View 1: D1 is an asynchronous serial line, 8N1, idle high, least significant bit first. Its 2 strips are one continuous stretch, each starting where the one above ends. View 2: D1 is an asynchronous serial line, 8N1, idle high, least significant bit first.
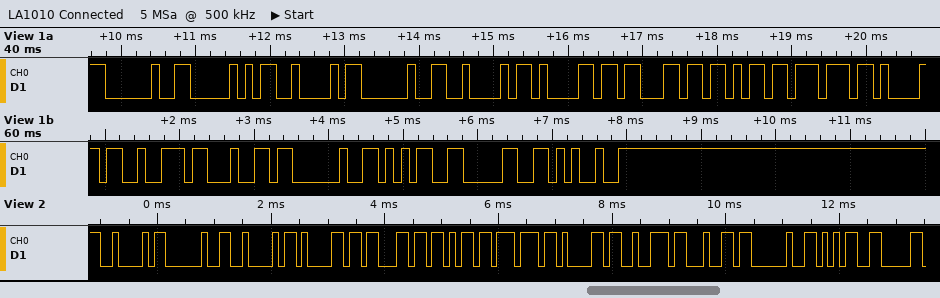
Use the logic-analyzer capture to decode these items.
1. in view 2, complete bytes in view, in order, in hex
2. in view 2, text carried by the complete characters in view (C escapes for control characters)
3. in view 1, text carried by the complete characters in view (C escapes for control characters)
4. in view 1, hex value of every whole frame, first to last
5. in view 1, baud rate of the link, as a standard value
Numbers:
42 20 42 61 63 6B 77 61 72 64 20 35
"B Backward 5"
" PB Backward 50%"
0x20 0x50 0x42 0x20 0x42 0x61 0x63 0x6B 0x77 0x61 0x72 0x64 0x20 0x35 0x30 0x25
9600 baud
